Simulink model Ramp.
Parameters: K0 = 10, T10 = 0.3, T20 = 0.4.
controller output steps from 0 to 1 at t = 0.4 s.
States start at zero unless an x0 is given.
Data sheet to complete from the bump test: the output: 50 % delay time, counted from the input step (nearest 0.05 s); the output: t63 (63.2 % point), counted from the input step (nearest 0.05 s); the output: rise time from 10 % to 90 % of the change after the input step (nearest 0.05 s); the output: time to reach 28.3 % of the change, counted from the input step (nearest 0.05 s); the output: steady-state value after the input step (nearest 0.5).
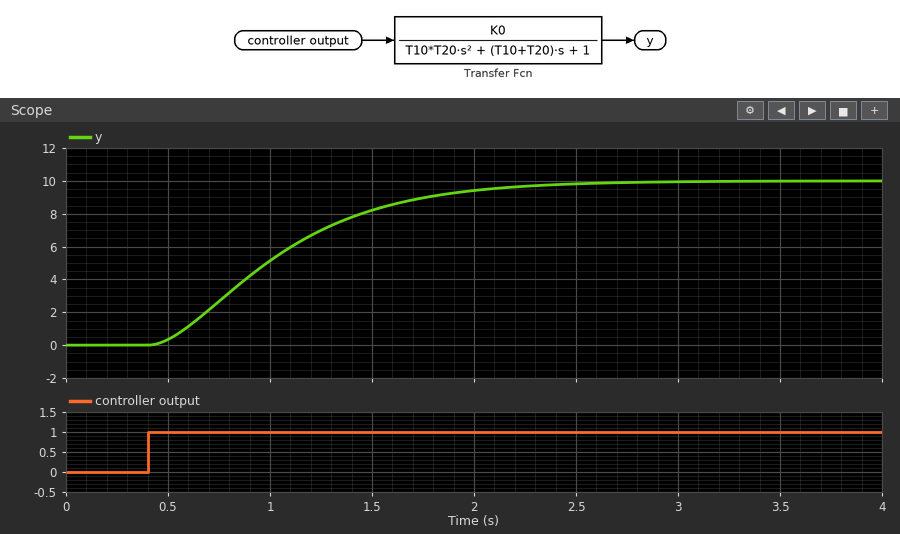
0.60 s
0.75 s
1.20 s
0.35 s
10.0
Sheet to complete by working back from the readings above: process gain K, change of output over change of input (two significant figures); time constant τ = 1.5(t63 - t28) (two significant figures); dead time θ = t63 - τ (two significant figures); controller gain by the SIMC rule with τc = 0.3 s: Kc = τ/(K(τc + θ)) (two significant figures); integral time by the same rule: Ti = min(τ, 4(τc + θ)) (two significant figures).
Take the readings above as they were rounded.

10
0.60 s
0.15 s
0.13
0.60 s
